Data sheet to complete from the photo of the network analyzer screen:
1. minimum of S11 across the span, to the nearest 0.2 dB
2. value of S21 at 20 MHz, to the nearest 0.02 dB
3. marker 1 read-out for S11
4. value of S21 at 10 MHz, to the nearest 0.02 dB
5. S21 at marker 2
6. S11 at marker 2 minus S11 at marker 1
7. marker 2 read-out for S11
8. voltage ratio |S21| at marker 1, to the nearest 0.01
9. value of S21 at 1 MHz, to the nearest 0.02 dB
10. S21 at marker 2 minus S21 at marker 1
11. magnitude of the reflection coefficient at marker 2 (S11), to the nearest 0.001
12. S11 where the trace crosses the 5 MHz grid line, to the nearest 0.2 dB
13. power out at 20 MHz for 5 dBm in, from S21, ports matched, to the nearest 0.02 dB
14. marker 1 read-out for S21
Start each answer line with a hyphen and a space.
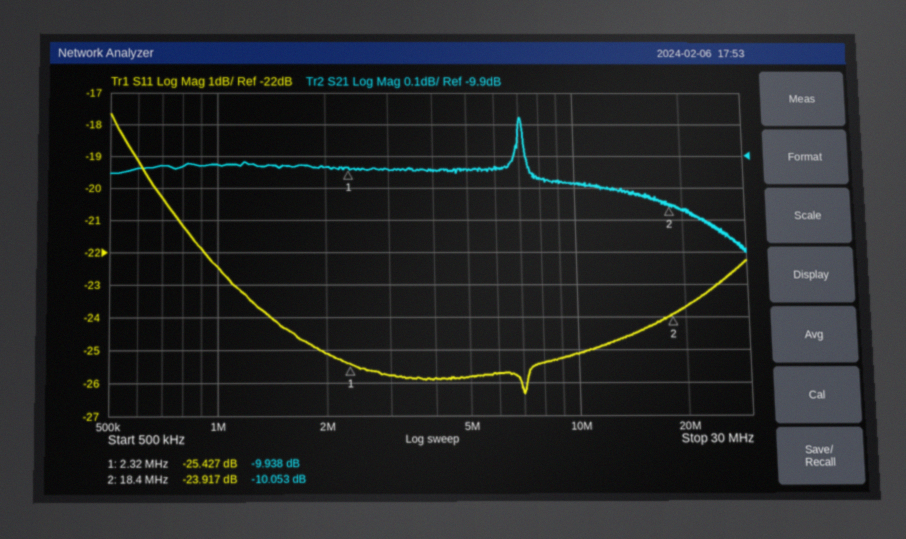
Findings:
- -26.4 dB
- -10.06 dB
- -25.427 dB
- -9.98 dB
- -10.053 dB
- 1.510 dB
- -23.917 dB
- 0.32
- -9.92 dB
- -0.115 dB
- 0.064
- -25.8 dB
- -5.06 dBm
- -9.938 dB
